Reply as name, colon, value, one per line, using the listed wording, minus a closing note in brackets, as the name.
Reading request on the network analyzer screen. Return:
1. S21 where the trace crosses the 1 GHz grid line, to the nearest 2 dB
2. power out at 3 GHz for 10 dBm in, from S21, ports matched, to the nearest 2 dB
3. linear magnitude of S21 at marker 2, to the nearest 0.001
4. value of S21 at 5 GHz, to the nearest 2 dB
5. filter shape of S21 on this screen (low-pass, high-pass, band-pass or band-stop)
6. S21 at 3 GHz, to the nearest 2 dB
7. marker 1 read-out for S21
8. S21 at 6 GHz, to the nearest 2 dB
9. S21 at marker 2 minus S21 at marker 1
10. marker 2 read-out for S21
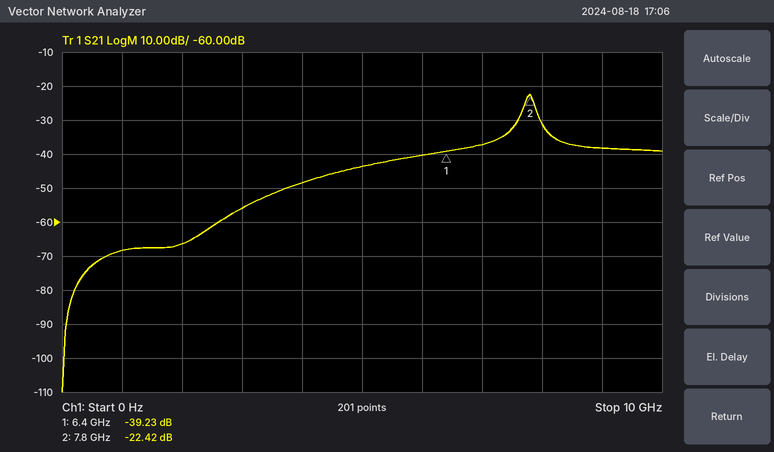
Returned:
S21 where the trace crosses the 1 GHz grid line, to the nearest 2 dB: -68 dB
power out at 3 GHz for 10 dBm in, from S21, ports matched, to the nearest 2 dB: -46 dBm
linear magnitude of S21 at marker 2, to the nearest 0.001: 0.076
value of S21 at 5 GHz, to the nearest 2 dB: -44 dB
filter shape of S21 on this screen: band-pass
S21 at 3 GHz, to the nearest 2 dB: -56 dB
marker 1 read-out for S21: -39.23 dB
S21 at 6 GHz, to the nearest 2 dB: -40 dB
S21 at marker 2 minus S21 at marker 1: 16.81 dB
marker 2 read-out for S21: -22.42 dB
